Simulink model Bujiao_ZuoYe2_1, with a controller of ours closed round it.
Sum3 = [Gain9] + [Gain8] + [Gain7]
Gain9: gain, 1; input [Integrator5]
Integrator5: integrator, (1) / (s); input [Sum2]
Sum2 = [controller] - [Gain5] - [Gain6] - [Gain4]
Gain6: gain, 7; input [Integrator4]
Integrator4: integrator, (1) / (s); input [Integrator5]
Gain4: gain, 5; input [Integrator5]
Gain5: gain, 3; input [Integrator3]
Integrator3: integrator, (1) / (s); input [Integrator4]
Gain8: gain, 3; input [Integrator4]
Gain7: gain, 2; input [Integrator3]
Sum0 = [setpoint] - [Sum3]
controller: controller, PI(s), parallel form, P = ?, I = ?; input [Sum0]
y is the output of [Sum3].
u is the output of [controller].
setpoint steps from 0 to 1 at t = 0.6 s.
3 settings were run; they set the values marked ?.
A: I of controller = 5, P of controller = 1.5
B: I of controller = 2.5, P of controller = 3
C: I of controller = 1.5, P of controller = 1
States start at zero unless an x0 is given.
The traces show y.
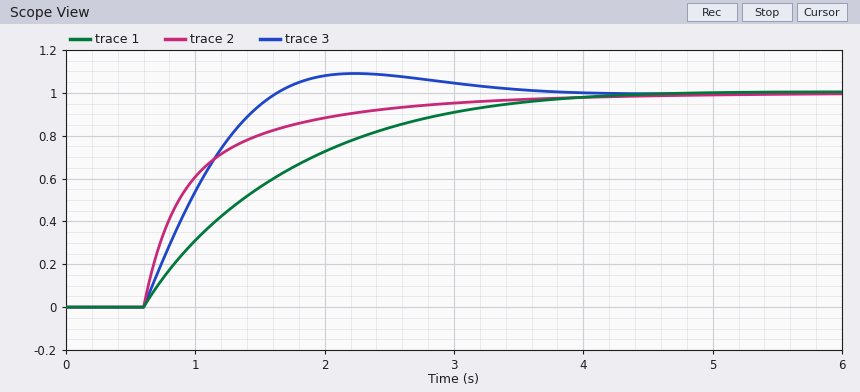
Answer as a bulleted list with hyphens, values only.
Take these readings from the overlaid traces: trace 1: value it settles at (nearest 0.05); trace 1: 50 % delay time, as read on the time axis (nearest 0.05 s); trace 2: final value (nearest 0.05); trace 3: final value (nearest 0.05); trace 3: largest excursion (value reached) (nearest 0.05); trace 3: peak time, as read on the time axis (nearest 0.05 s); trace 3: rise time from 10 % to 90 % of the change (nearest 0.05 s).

- 1.00
- 1.35 s
- 1.00
- 1.00
- 1.10
- 2.25 s
- 0.75 s
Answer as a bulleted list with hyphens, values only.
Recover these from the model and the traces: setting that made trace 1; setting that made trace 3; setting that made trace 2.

- C
- A
- B
